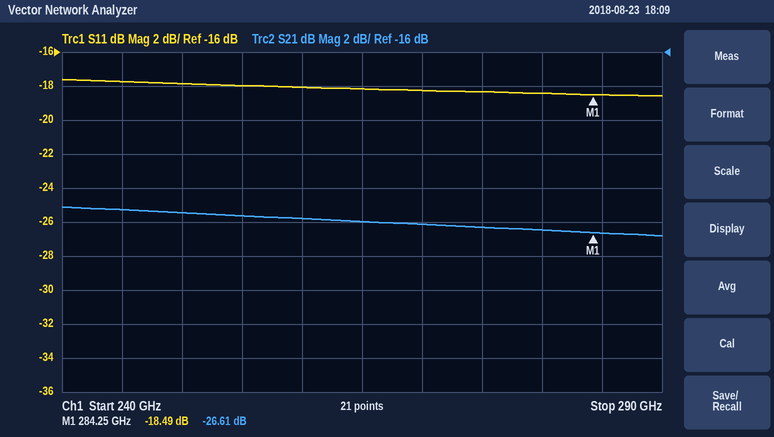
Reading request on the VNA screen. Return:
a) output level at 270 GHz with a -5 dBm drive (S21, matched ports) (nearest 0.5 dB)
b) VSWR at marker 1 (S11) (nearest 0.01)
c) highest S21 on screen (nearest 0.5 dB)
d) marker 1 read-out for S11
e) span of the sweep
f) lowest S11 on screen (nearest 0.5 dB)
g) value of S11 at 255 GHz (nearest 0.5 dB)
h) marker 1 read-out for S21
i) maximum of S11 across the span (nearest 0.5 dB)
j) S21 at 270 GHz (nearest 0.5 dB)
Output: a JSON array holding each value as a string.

["-31.0 dBm", "1.27", "-25.0 dB", "-18.49 dB", "50 GHz", "-18.5 dB", "-18.0 dB", "-26.61 dB", "-17.5 dB", "-26.0 dB"]
